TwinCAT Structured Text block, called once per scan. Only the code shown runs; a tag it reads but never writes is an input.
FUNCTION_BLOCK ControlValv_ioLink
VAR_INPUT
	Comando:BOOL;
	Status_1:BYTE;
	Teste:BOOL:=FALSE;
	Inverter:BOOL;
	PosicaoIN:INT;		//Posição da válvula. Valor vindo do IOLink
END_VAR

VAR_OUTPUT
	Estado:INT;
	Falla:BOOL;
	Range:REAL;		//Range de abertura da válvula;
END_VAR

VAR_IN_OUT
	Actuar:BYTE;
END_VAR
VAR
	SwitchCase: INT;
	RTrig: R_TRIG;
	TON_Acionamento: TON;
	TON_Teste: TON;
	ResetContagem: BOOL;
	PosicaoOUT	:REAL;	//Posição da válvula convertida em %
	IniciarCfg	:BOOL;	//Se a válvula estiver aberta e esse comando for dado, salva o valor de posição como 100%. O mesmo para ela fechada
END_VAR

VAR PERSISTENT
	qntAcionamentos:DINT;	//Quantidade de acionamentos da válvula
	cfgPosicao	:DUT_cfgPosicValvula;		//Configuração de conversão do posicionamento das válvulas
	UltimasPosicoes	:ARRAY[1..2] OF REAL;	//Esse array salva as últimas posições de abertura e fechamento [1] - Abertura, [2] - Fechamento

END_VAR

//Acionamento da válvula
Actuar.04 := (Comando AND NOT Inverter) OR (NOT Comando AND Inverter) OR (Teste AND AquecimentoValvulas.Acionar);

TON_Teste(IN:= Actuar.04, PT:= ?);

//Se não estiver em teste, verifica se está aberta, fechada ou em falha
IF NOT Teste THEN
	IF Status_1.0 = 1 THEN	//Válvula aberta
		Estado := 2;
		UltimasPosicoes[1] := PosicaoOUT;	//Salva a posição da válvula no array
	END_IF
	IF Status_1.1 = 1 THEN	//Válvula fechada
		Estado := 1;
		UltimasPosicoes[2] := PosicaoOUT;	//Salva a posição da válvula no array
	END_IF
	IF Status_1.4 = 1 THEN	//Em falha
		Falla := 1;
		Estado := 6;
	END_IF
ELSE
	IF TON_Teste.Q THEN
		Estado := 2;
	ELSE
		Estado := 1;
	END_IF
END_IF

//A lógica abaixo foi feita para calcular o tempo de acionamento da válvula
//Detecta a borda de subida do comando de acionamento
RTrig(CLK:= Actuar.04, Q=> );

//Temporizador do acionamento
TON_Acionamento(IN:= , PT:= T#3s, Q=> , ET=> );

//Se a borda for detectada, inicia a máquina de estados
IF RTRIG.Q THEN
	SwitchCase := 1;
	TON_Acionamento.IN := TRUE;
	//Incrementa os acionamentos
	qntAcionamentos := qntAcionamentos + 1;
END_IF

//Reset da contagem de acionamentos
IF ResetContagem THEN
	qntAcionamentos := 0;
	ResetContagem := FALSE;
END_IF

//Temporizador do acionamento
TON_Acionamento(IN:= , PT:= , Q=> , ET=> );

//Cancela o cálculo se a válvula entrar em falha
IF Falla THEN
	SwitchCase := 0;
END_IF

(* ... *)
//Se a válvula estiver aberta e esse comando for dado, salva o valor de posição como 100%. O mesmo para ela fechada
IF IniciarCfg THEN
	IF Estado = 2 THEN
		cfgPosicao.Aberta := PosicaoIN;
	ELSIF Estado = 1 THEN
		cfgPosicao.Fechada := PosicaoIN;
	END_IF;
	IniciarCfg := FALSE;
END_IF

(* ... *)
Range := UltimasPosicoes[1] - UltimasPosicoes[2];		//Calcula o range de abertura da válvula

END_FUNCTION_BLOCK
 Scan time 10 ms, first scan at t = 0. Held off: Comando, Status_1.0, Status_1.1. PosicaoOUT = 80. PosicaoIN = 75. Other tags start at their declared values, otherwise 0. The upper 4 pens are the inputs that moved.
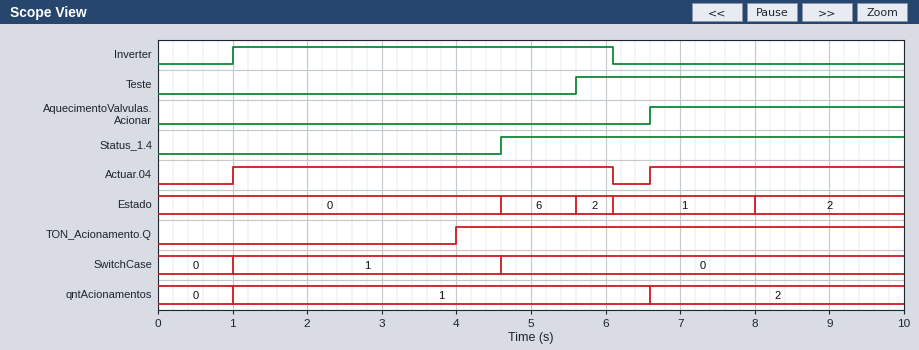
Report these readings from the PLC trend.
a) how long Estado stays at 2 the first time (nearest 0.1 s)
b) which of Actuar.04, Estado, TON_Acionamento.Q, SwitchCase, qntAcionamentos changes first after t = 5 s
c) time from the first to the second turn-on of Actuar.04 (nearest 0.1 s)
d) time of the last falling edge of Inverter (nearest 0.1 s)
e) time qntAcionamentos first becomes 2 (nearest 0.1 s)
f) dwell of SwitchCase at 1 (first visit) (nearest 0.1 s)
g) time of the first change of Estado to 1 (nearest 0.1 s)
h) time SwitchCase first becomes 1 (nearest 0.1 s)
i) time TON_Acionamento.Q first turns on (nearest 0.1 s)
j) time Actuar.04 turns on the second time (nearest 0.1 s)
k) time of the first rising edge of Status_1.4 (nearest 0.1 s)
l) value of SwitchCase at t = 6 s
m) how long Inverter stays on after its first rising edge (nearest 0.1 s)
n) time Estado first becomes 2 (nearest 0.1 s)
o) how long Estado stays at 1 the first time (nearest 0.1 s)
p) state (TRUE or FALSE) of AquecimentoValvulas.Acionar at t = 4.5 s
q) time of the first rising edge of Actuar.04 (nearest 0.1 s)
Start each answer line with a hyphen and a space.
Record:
- 0.5 s
- Estado
- 5.6 s
- 6.1 s
- 6.6 s
- 3.6 s
- 6.1 s
- 1.0 s
- 4.0 s
- 6.6 s
- 4.6 s
- 0
- 5.1 s
- 5.6 s
- 1.9 s
- FALSE
- 1.0 s
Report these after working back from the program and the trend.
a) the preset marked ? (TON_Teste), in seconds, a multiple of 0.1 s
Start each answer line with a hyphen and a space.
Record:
- 1.4 s
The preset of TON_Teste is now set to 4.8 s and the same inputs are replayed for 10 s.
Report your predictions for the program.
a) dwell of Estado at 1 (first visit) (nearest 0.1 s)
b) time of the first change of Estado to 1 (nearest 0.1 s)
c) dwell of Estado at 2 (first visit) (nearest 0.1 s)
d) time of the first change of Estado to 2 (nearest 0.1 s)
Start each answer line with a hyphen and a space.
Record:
- 0.2 s
- 5.6 s
- 0.3 s
- 5.8 s
